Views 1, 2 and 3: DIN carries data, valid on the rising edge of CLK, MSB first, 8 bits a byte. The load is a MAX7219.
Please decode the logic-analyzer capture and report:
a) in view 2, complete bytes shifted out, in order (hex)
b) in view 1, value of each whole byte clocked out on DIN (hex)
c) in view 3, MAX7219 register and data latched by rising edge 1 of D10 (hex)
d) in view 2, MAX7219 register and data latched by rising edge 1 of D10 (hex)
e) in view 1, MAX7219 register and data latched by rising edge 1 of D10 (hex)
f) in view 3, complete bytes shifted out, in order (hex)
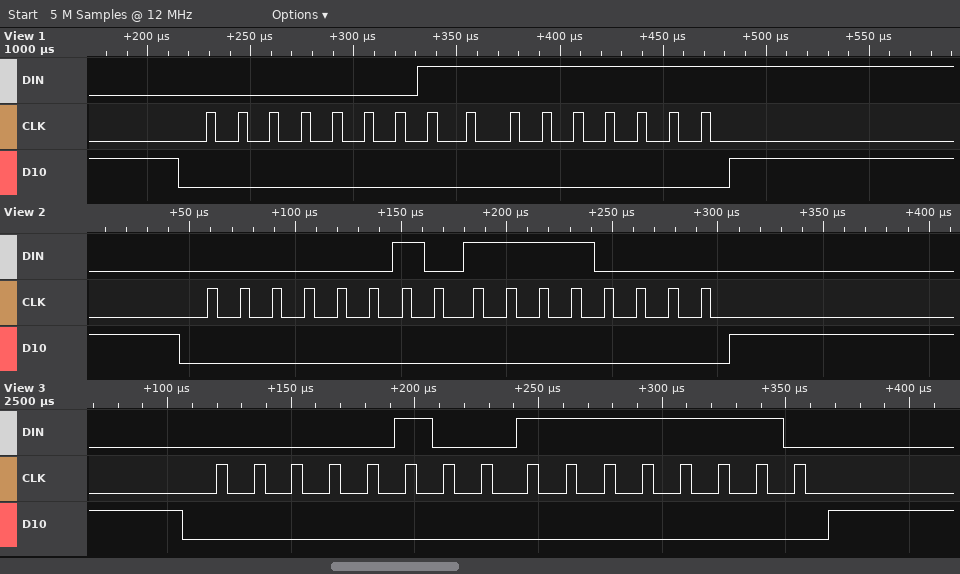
02 F0
01 FF
register 0x4, data 0xFE
register 0x2, data 0xF0
register 0x1, data 0xFF
0x04 0xFE
